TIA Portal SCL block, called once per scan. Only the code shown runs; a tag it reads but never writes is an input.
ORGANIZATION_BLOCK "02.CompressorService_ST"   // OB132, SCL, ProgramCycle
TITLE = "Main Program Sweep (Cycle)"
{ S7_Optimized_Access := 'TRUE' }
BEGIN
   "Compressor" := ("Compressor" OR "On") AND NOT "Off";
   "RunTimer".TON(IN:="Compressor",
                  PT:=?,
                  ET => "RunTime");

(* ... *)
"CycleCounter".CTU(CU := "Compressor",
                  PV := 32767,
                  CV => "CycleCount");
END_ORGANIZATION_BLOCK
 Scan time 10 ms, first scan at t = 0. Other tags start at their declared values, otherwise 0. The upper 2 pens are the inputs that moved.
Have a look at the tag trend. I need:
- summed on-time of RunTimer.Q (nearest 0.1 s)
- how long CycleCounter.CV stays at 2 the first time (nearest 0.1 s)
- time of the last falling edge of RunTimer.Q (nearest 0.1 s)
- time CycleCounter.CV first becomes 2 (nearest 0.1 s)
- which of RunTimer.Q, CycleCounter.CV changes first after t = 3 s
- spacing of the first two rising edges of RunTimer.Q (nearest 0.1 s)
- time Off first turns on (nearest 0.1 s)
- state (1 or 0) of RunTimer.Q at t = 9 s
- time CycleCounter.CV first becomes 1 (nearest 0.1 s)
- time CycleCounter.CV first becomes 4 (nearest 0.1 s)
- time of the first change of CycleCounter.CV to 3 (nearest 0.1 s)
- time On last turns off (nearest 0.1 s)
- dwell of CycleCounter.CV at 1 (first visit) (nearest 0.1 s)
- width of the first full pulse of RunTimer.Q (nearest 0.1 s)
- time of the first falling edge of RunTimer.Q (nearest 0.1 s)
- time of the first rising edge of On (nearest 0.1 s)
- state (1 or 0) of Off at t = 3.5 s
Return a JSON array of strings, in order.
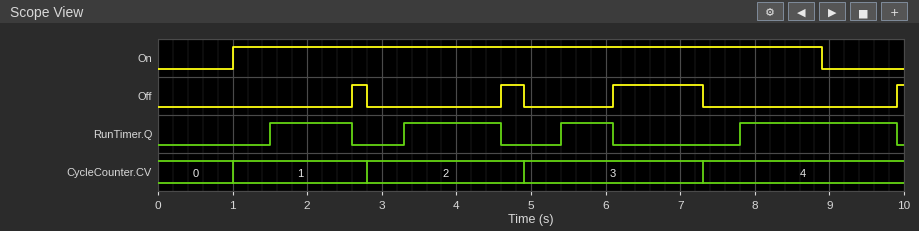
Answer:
["5.2 s", "2.1 s", "9.9 s", "2.8 s", "RunTimer.Q", "1.8 s", "2.6 s", "1", "1.0 s", "7.3 s", "4.9 s", "8.9 s", "1.8 s", "1.1 s", "2.6 s", "1.0 s", "0"]
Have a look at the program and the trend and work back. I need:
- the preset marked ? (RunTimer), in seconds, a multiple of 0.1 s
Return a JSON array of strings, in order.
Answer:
["0.5 s"]
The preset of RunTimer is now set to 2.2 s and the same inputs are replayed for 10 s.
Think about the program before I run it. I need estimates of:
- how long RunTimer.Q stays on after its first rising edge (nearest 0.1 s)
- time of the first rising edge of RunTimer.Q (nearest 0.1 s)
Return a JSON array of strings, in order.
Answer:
["0.4 s", "9.5 s"]
